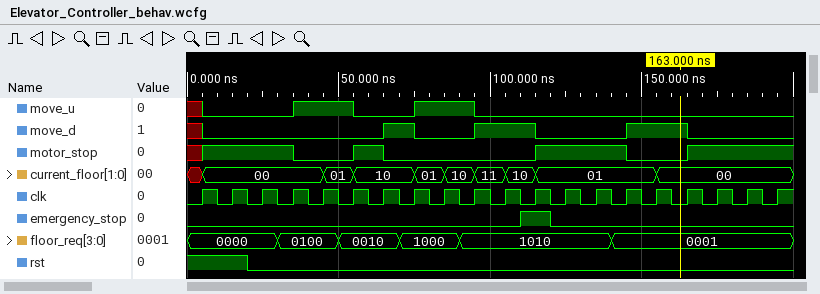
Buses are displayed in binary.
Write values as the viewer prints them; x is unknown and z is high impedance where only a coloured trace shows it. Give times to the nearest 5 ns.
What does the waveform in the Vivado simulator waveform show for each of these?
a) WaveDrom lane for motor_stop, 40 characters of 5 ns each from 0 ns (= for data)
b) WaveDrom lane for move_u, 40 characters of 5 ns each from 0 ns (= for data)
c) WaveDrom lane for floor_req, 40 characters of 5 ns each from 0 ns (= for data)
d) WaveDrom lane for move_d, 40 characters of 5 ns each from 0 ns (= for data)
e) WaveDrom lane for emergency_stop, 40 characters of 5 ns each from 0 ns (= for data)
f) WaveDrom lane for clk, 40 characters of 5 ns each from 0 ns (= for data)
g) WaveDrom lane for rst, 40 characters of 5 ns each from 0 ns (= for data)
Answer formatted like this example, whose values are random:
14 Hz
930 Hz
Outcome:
{name: 'motor_stop', wave: 'x1.....0...1.0.........1.....0...1......'}
{name: 'move_u', wave: 'x0.....1...0...1...0....................'}
{name: 'floor_req', wave: '=.....=...=...=...=.........=...........', data: '0000 0100 0010 1000 1010 0001'}
{name: 'move_d', wave: 'x0...........1.0...1...0.....1...0......'}
{name: 'emergency_stop', wave: '0.....................1.0...............'}
{name: 'clk', wave: '0101010101010101010101010101010101010101'}
{name: 'rst', wave: '1...0...................................'}
